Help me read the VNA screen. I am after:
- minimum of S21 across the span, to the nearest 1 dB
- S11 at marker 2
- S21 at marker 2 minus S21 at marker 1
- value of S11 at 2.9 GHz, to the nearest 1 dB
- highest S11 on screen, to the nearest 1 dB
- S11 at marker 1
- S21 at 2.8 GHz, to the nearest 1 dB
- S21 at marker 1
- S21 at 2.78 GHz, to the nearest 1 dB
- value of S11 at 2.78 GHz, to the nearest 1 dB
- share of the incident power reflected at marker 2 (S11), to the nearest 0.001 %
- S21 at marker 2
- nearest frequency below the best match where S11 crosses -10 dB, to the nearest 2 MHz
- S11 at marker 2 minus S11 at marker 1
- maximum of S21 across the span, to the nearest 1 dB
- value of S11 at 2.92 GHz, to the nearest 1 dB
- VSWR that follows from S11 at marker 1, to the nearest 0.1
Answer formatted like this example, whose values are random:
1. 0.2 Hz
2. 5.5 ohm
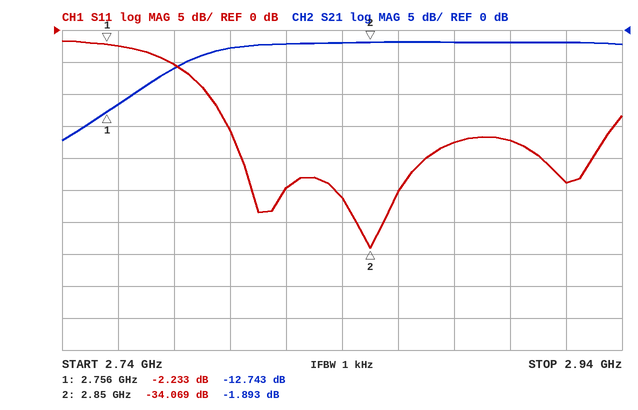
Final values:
1. -17 dB
2. -34.069 dB
3. 10.850 dB
4. -17 dB
5. -2 dB
6. -2.233 dB
7. -3 dB
8. -12.743 dB
9. -6 dB
10. -5 dB
11. 0.039 %
12. -1.893 dB
13. 2.792 GHz
14. -31.836 dB
15. -2 dB
16. -24 dB
17. 7.8
